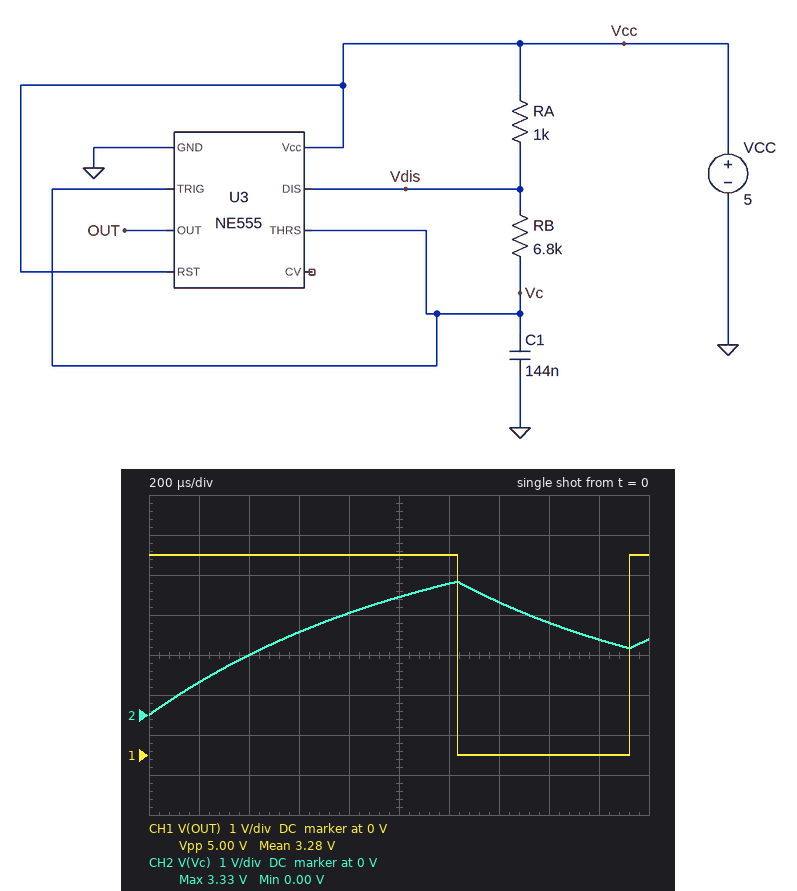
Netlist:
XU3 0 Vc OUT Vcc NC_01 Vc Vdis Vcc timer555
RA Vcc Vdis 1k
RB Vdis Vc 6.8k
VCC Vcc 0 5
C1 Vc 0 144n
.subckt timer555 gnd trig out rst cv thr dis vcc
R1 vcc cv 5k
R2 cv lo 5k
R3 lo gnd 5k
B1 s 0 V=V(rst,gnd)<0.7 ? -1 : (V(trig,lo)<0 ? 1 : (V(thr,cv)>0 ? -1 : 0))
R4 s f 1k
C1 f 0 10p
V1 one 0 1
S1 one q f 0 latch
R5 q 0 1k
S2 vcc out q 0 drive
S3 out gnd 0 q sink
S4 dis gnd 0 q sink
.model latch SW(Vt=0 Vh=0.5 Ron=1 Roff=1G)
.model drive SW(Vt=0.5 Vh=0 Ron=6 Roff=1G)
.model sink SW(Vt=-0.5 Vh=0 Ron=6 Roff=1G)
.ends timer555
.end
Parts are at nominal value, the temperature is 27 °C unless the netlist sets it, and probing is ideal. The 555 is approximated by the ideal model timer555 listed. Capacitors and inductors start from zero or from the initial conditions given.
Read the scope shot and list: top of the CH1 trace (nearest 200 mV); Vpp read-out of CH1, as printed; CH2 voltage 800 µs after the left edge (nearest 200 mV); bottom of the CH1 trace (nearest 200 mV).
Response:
5.0 V
5.00 V
2.6 V
0 V
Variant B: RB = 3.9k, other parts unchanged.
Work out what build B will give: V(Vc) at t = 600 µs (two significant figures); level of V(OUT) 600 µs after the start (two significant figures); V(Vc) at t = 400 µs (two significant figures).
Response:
2.9 V
5.0 V
2.2 V
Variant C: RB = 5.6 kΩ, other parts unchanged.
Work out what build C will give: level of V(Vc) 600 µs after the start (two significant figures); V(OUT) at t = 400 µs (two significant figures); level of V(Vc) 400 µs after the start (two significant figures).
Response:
2.3 V
5.0 V
1.7 V
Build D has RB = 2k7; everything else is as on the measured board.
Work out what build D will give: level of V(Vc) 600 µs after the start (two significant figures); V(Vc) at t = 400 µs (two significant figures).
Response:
3.2 V
2.6 V
